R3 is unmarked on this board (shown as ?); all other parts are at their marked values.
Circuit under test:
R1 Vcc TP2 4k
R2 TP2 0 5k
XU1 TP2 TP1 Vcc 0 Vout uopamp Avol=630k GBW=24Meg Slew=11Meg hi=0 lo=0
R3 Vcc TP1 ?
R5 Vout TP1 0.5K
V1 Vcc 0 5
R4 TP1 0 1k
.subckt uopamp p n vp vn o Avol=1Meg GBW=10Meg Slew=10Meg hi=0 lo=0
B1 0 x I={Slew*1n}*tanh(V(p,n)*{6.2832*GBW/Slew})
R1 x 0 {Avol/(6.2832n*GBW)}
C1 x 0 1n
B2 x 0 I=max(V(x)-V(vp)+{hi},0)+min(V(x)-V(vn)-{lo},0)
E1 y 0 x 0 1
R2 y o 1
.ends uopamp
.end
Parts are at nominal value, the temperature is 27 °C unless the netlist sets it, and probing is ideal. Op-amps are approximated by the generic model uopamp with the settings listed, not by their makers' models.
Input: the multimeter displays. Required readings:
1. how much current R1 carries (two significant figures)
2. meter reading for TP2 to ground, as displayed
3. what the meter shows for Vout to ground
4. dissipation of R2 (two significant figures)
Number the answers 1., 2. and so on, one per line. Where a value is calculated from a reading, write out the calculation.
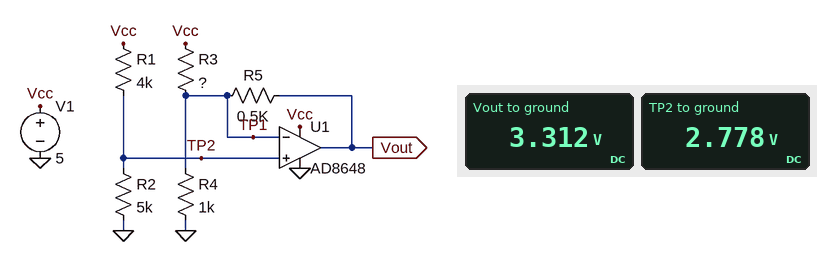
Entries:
1. (5 V - 2.778 V) / 4 kΩ = 560 µA
2. 2.778 V
3. 3.312 V
4. (2.778 V)^2 / 5 kΩ = 1.5 mW
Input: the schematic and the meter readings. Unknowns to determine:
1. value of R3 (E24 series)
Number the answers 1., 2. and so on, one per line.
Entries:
1. 1.3 kΩ
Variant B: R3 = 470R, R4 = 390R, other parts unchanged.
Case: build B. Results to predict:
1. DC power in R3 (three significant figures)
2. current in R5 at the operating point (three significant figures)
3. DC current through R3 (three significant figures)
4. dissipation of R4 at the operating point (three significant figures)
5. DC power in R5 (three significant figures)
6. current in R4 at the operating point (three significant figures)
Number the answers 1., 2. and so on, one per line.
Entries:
1. 10.5 mW
2. 2.39 mA
3. 4.73 mA
4. 19.8 mW
5. 2.87 mW
6. 7.12 mA
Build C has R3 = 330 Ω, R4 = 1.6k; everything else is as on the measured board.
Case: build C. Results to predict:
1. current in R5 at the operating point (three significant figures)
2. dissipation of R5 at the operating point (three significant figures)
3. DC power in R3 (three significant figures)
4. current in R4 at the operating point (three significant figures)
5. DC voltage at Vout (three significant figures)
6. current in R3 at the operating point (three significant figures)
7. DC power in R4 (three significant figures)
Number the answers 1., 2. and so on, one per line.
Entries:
1. 5.00 mA
2. 12.5 mW
3. 15.0 mW
4. 1.74 mA
5. 279 mV
6. 6.73 mA
7. 4.82 mW
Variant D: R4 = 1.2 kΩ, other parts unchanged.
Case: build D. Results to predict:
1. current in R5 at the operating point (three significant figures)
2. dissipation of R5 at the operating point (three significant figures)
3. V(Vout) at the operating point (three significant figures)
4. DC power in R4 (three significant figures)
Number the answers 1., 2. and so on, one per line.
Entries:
1. 605 µA
2. 183 µW
3. 3.08 V
4. 6.43 mW
